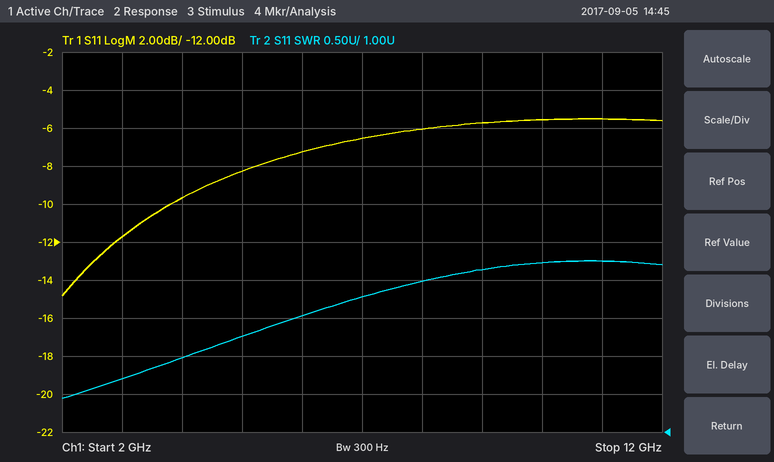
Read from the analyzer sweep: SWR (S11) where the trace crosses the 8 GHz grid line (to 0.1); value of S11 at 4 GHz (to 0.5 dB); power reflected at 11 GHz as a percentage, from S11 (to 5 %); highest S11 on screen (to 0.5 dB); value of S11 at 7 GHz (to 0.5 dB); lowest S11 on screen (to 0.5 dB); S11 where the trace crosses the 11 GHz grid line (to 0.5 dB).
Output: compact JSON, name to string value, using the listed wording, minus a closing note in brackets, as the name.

{"SWR (S11) where the trace crosses the 8 GHz grid line": "3.0", "value of S11 at 4 GHz": "-9.5 dB", "power reflected at 11 GHz as a percentage, from S11": "30 %", "highest S11 on screen": "-5.5 dB", "value of S11 at 7 GHz": "-6.5 dB", "lowest S11 on screen": "-15.0 dB", "S11 where the trace crosses the 11 GHz grid line": "-5.5 dB"}
